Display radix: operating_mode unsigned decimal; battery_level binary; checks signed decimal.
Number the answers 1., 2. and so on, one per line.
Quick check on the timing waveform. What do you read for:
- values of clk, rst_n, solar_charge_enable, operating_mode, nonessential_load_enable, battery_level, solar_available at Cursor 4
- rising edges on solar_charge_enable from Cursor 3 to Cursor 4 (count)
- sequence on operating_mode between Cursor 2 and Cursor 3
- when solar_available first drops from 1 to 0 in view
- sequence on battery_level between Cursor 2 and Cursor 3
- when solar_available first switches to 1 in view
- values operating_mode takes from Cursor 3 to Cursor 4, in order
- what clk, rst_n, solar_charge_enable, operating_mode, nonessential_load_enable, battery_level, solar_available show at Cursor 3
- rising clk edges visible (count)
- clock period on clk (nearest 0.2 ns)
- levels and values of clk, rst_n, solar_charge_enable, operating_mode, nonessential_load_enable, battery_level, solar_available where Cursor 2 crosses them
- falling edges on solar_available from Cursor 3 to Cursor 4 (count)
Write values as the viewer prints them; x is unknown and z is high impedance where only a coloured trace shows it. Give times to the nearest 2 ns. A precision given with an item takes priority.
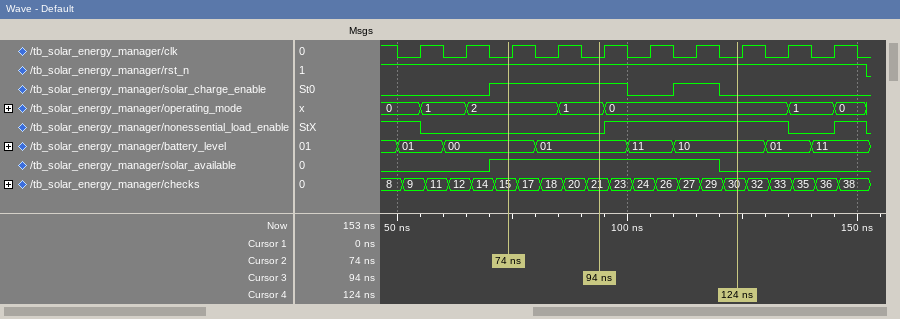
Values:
1. clk=0, rst_n=1, solar_charge_enable=0, operating_mode=0, nonessential_load_enable=1, battery_level=10, solar_available=0
2. 1
3. 2, 1
4. 120 ns
5. 00, 01
6. 70 ns
7. 1, 0
8. clk=0, rst_n=1, solar_charge_enable=1, operating_mode=1, nonessential_load_enable=0, battery_level=01, solar_available=1
9. 10
10. 10 ns
11. clk=0, rst_n=1, solar_charge_enable=1, operating_mode=2, nonessential_load_enable=0, battery_level=00, solar_available=1
12. 1
